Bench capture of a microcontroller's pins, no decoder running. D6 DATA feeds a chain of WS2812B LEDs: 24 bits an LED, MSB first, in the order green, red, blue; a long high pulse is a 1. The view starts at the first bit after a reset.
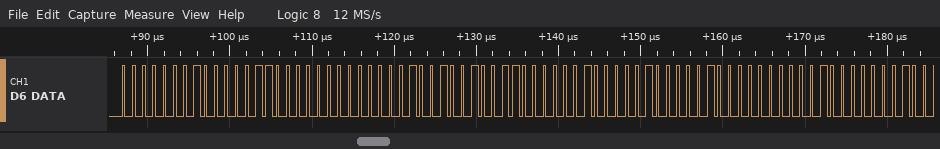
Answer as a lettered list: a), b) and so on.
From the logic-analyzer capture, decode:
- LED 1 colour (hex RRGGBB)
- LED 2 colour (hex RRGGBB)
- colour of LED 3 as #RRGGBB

a) #060100
b) #260904
c) #401008
